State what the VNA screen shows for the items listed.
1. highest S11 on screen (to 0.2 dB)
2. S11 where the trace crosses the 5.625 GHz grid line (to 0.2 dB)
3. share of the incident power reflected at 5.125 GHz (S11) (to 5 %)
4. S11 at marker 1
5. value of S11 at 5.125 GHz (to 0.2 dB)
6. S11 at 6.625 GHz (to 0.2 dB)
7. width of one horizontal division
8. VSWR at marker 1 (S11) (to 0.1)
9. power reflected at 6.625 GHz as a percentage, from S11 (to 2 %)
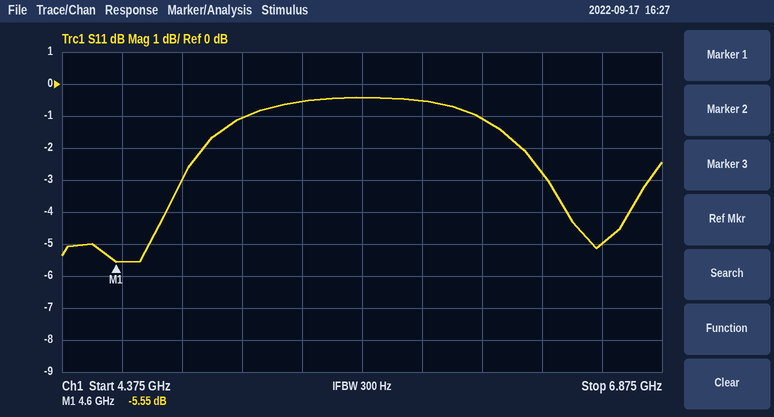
-0.4 dB
-0.4 dB
80 %
-5.55 dB
-1.0 dB
-5.0 dB
250 MHz
3.2
32 %
